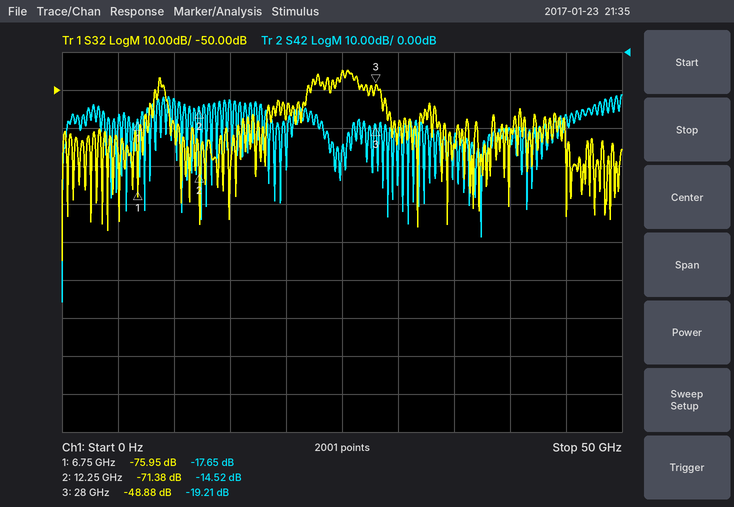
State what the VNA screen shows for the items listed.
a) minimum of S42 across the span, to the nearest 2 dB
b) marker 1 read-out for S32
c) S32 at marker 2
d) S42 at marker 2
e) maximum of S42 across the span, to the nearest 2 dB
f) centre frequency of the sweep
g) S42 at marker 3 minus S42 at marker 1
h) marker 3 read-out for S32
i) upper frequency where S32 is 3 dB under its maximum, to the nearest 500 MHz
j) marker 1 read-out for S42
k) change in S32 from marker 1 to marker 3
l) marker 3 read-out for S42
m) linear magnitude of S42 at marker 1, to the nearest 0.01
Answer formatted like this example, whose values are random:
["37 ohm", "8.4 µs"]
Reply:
["-66 dB", "-75.95 dB", "-71.38 dB", "-14.52 dB", "-12 dB", "25 GHz", "-1.56 dB", "-48.88 dB", "26.5 GHz", "-17.65 dB", "27.07 dB", "-19.21 dB", "0.13"]
